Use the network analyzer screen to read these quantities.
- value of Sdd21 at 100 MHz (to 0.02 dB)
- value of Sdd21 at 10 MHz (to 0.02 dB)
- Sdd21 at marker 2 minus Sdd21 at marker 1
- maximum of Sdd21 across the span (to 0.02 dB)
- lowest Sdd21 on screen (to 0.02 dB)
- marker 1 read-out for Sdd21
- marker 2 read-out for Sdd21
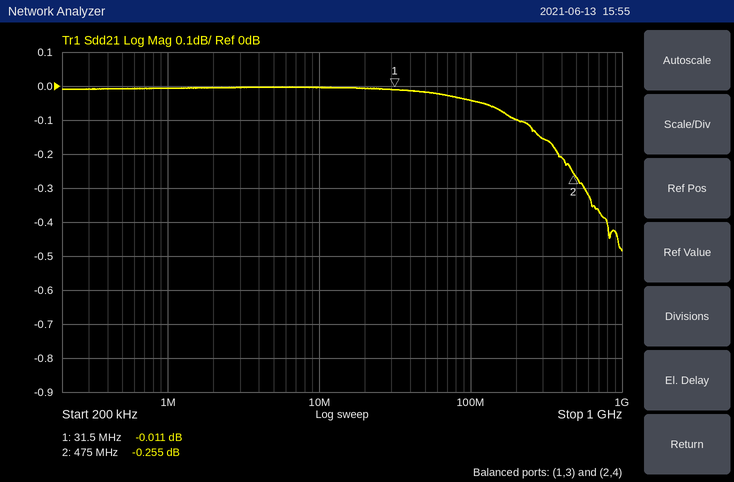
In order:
-0.04 dB
0.00 dB
-0.244 dB
0.00 dB
-0.48 dB
-0.011 dB
-0.255 dB
